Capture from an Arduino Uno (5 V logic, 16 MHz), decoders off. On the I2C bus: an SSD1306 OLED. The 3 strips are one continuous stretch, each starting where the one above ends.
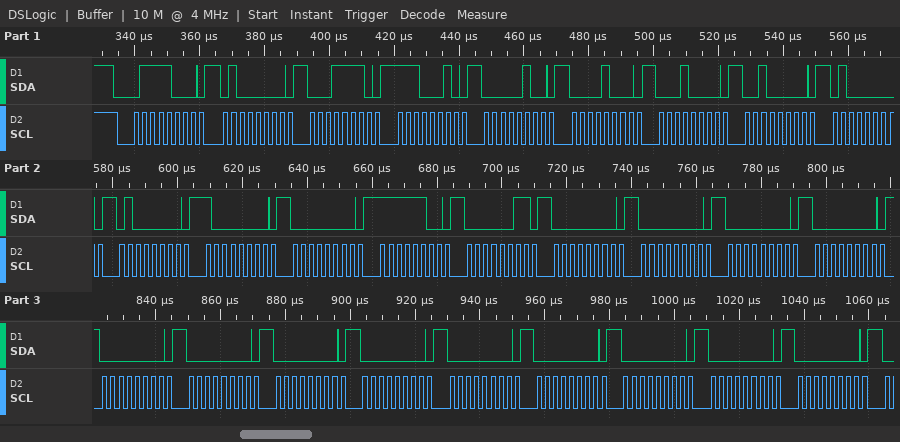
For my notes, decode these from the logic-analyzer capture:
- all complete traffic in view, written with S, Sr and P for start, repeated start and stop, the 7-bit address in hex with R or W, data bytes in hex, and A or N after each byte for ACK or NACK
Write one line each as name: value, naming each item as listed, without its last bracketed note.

all complete traffic in view, written with S, Sr and P for start, repeated start and stop, the 7-bit address in hex with R or W, data bytes in hex, and A or N after each byte for ACK or NACK: S 3CW A 40 A 1E A E2 A 04 A 08 A 10 A 20 A 40 A 40 A 80 A 00 A FC A 03 A 00 A 00 A 00 A 00 A 00 A 00 A 00 A 00 A 00 A 00 A 00 A 00 A 00 A
